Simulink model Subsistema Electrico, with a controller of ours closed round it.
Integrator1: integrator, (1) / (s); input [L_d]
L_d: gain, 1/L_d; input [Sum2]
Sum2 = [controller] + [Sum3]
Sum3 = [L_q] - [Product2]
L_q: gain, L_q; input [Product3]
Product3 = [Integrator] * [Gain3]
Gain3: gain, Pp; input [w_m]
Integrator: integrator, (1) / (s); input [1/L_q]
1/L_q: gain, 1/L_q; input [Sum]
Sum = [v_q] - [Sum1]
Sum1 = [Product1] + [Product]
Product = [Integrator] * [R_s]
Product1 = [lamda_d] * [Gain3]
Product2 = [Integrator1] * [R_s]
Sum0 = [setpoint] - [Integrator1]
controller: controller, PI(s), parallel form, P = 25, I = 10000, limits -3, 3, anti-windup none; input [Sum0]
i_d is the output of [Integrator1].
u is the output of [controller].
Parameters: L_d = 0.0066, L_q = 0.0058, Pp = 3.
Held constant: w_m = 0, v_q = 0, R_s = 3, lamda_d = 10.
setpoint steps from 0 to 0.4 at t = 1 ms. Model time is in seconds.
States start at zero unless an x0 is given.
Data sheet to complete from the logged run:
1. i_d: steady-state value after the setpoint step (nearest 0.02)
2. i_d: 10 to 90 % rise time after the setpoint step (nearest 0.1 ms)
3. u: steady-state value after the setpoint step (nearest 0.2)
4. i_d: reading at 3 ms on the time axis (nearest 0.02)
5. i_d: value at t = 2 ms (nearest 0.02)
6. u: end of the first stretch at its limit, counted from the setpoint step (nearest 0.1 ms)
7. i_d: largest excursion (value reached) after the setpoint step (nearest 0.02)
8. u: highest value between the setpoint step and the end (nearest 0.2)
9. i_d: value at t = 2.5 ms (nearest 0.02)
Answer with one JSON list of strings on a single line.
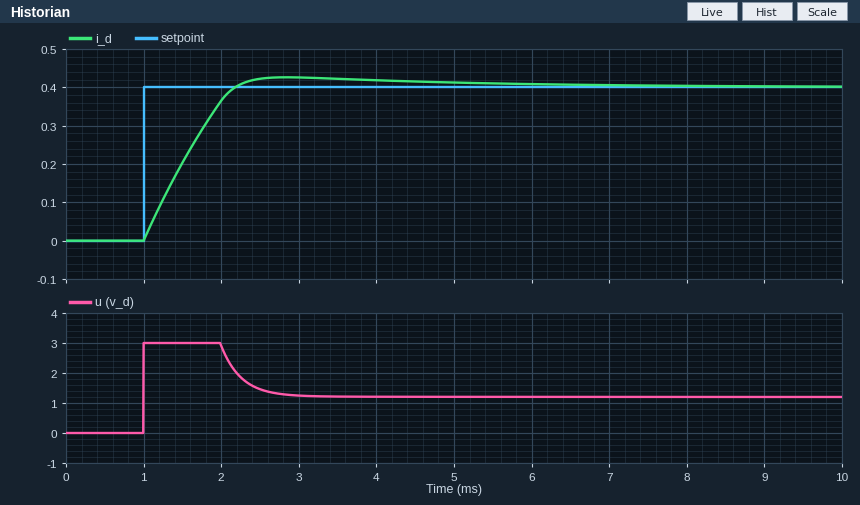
["0.40", "0.9 ms", "1.2", "0.42", "0.36", "1.0 ms", "0.42", "3.0", "0.42"]
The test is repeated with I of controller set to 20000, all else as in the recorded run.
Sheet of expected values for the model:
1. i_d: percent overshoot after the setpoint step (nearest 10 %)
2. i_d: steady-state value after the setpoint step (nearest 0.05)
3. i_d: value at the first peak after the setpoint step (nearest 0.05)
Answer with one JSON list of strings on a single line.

["20 %", "0.40", "0.50"]
